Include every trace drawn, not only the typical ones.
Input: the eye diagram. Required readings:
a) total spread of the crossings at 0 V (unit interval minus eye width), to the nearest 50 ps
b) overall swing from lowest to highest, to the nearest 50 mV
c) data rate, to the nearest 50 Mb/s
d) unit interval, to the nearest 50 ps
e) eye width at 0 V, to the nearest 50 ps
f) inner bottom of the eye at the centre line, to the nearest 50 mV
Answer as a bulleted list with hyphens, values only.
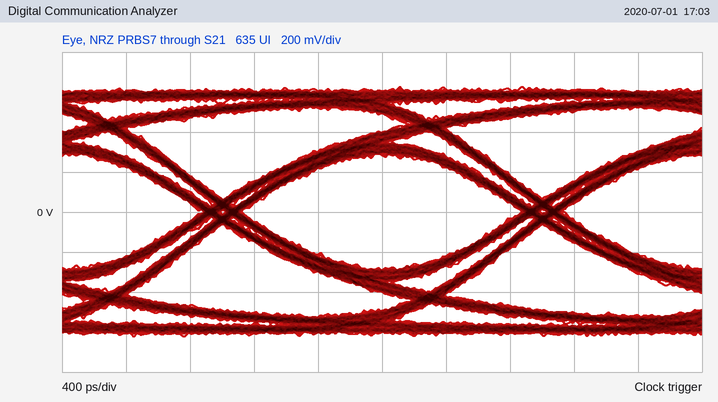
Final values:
- 250 ps
- 1.25 V
- 500 Mb/s
- 2.00 ns
- 1.75 ns
- -300 mV
